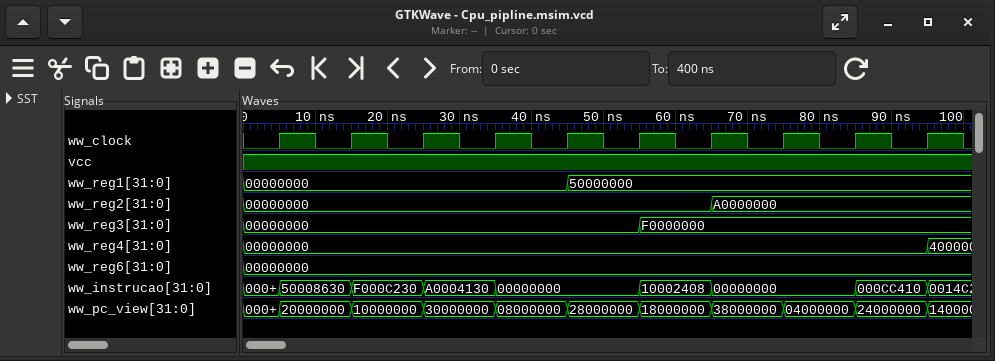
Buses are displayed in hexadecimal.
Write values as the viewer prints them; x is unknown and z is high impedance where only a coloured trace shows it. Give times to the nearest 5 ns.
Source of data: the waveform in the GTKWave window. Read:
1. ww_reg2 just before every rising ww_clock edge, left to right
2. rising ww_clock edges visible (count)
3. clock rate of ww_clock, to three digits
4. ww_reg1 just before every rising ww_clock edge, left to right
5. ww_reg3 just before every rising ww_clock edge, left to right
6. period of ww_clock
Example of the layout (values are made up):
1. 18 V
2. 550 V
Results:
1. 00000000, 00000000, 00000000, 00000000, 00000000, 00000000, 00000000, A0000000, A0000000, A0000000
2. 10
3. 100 MHz
4. 00000000, 00000000, 00000000, 00000000, 00000000, 50000000, 50000000, 50000000, 50000000, 50000000
5. 00000000, 00000000, 00000000, 00000000, 00000000, 00000000, F0000000, F0000000, F0000000, F0000000
6. 10 ns
